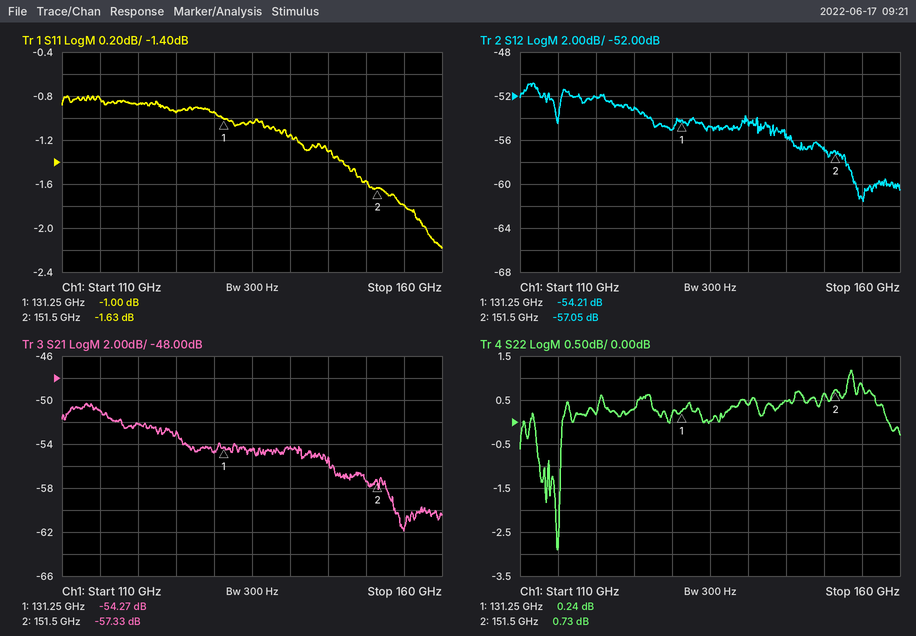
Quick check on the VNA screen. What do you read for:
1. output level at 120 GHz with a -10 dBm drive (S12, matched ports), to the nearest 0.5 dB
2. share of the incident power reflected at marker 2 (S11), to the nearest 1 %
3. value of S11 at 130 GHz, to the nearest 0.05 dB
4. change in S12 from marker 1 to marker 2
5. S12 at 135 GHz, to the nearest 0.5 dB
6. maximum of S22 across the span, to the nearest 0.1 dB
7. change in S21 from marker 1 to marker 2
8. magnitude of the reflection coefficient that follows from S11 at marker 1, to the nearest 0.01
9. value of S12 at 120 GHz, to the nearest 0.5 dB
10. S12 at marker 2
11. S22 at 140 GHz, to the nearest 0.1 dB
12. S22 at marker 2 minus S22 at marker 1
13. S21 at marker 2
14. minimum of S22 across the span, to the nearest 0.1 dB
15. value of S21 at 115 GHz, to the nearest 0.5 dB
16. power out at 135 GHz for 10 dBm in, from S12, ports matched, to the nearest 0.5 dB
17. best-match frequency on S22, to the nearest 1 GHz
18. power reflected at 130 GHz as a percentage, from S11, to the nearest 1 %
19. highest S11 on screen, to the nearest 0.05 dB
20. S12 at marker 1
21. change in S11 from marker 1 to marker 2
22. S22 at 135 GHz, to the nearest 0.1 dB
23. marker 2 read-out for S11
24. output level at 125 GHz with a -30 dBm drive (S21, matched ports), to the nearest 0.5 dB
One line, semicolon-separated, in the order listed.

-62.0 dBm; 69 %; -0.95 dB; -2.84 dB; -55.0 dB; 1.2 dB; -3.06 dB; 0.89; -52.0 dB; -57.05 dB; 0.4 dB; 0.49 dB; -57.33 dB; -2.9 dB; -51.0 dB; -45.0 dBm; 115 GHz; 80 %; -0.80 dB; -54.21 dB; -0.63 dB; 0.0 dB; -1.63 dB; -83.0 dBm
